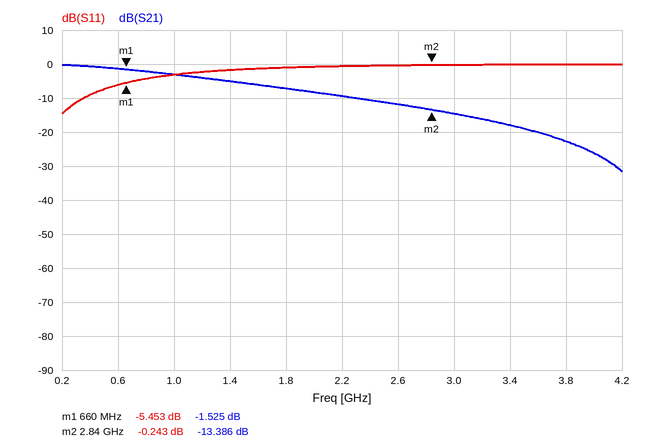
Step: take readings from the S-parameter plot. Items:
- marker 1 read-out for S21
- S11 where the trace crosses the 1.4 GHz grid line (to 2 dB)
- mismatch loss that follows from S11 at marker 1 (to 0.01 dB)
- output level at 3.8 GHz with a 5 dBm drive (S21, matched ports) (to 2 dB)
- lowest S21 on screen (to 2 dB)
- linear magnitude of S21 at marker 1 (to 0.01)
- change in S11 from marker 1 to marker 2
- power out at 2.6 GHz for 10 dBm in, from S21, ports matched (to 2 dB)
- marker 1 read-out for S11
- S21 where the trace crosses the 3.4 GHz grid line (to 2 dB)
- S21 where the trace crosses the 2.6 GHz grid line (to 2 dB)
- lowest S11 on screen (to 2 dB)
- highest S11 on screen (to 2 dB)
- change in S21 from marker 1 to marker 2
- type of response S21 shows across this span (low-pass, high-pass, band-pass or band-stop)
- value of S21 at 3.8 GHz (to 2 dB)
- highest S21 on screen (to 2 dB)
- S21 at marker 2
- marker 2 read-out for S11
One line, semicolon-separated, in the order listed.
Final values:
-1.525 dB; -2 dB; 1.46 dB; -18 dBm; -32 dB; 0.84; 5.210 dB; -2 dBm; -5.453 dB; -18 dB; -12 dB; -14 dB; 0 dB; -11.861 dB; low-pass; -22 dB; 0 dB; -13.386 dB; -0.243 dB
